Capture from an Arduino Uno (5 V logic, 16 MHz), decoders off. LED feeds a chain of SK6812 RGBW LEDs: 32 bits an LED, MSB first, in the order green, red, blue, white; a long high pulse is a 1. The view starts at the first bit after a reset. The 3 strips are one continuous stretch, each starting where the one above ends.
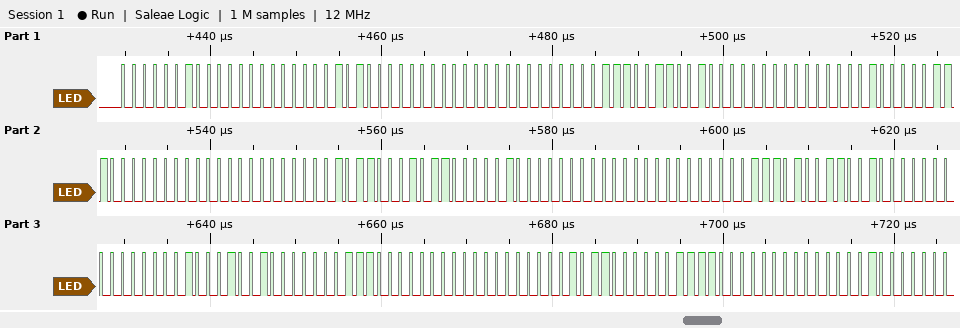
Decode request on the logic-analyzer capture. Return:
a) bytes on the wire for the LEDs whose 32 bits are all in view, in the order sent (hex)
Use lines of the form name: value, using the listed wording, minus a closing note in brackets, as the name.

bytes on the wire for the LEDs whose 32 bits are all in view, in the order sent: 02 00 0A 00 00 07 32 00 02 0E 00 00 0B 16 08 00 00 1D 32 00 02 24 07 00 00 2C 0F 00
